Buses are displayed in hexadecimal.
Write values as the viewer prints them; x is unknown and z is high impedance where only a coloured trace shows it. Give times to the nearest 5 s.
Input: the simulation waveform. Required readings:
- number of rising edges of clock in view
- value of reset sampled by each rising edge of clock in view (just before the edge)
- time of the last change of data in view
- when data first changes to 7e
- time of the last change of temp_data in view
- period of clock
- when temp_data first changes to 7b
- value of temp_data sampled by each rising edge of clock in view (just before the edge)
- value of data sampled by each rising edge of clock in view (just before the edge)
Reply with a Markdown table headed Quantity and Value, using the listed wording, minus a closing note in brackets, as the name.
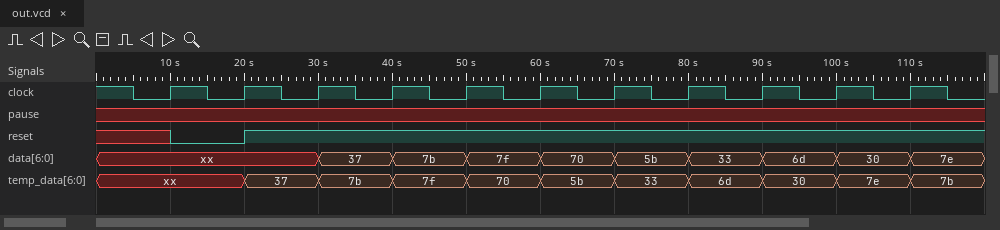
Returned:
| Quantity | Value |
|---|---|
| number of rising edges of clock in view | 11 |
| value of reset sampled by each rising edge of clock in view | x 0 1 1 1 1 1 1 1 1 1 |
| time of the last change of data in view | 110 s |
| when data first changes to 7e | 110 s |
| time of the last change of temp_data in view | 110 s |
| period of clock | 10 s |
| when temp_data first changes to 7b | 30 s |
| value of temp_data sampled by each rising edge of clock in view | xx, xx, 37, 7b, 7f, 70, 5b, 33, 6d, 30, 7e |
| value of data sampled by each rising edge of clock in view | xx, xx, xx, 37, 7b, 7f, 70, 5b, 33, 6d, 30 |
